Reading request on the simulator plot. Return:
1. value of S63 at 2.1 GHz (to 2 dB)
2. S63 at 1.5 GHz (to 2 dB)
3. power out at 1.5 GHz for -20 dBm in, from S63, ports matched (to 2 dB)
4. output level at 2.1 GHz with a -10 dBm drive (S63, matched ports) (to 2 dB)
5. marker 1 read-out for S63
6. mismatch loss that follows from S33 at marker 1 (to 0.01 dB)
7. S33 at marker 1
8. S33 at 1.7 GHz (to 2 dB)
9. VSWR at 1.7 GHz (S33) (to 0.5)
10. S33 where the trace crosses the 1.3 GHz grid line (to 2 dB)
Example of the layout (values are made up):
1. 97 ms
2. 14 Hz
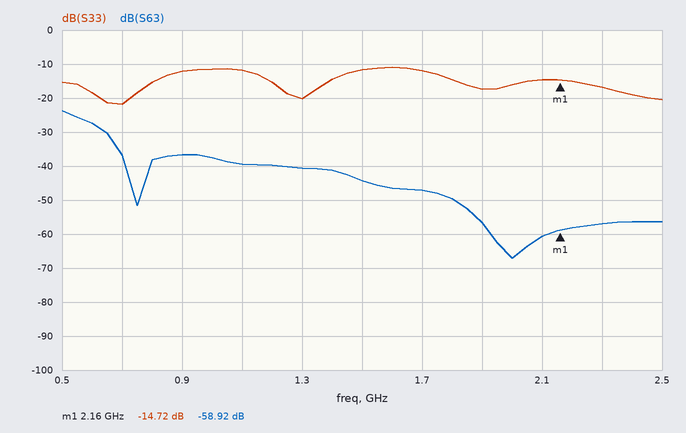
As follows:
1. -60 dB
2. -44 dB
3. -64 dBm
4. -70 dBm
5. -58.92 dB
6. 0.15 dB
7. -14.72 dB
8. -12 dB
9. 1.5
10. -20 dB
